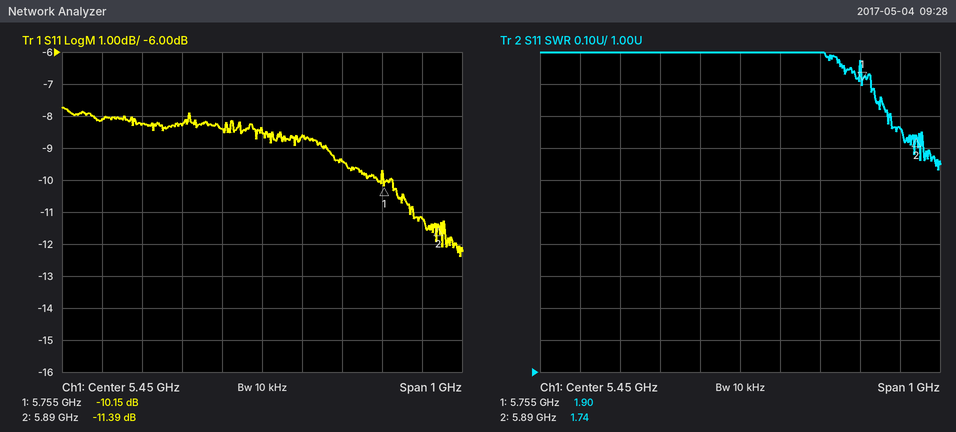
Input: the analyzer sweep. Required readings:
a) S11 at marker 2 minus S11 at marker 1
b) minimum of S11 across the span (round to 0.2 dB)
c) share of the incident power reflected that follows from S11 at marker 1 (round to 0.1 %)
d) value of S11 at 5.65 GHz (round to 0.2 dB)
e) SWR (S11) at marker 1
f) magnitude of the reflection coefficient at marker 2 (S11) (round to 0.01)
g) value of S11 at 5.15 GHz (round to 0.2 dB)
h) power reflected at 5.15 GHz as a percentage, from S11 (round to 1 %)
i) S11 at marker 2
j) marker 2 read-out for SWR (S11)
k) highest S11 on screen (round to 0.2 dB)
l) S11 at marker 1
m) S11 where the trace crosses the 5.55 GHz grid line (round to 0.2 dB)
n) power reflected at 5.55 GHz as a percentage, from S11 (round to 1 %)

-1.24 dB
-12.4 dB
9.7 %
-9.4 dB
1.90
0.27
-8.2 dB
15 %
-11.39 dB
1.74
-7.8 dB
-10.15 dB
-8.6 dB
14 %
